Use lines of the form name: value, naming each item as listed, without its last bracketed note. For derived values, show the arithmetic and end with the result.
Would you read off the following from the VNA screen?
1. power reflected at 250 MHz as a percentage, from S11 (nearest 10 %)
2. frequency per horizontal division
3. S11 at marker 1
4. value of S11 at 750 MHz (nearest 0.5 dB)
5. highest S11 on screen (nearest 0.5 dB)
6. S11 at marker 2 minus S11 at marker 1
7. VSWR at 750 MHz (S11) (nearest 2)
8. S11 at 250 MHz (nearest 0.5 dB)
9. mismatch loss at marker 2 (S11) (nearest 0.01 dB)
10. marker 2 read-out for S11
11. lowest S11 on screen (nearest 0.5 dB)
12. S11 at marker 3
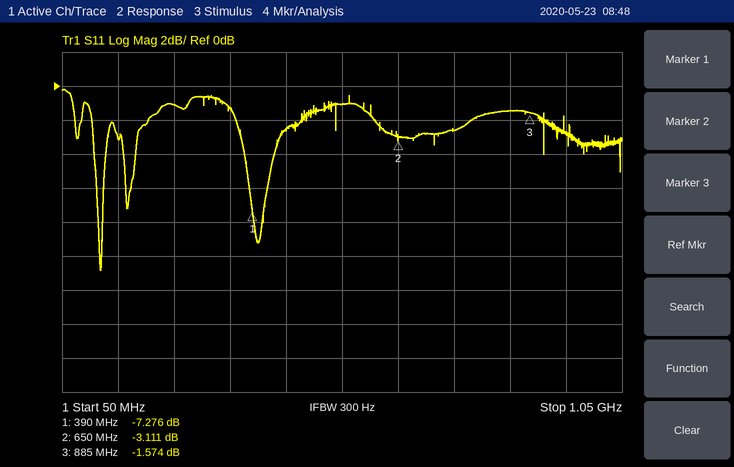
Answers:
power reflected at 250 MHz as a percentage, from S11: 10^(-1/10) ≈ 79.4 %, so 80 % to the nearest 10 %
frequency per horizontal division: 100 MHz
S11 at marker 1: -7.276 dB
value of S11 at 750 MHz: -2.5 dB
highest S11 on screen: 0.0 dB
S11 at marker 2 minus S11 at marker 1: -3.111 − (-7.276) = 4.165 dB
VSWR at 750 MHz (S11): |Γ| = 10^(-2.5/20) = 0.7499; VSWR = (1 + 0.7499)/(1 − 0.7499) ≈ 7.00, so 6 to the nearest 2
S11 at 250 MHz: -1.0 dB
mismatch loss at marker 2 (S11): −10 log10(1 − 10^(-3.111/10)) ≈ 2.91 dB
marker 2 read-out for S11: -3.111 dB
lowest S11 on screen: -11.0 dB
S11 at marker 3: -1.574 dB
